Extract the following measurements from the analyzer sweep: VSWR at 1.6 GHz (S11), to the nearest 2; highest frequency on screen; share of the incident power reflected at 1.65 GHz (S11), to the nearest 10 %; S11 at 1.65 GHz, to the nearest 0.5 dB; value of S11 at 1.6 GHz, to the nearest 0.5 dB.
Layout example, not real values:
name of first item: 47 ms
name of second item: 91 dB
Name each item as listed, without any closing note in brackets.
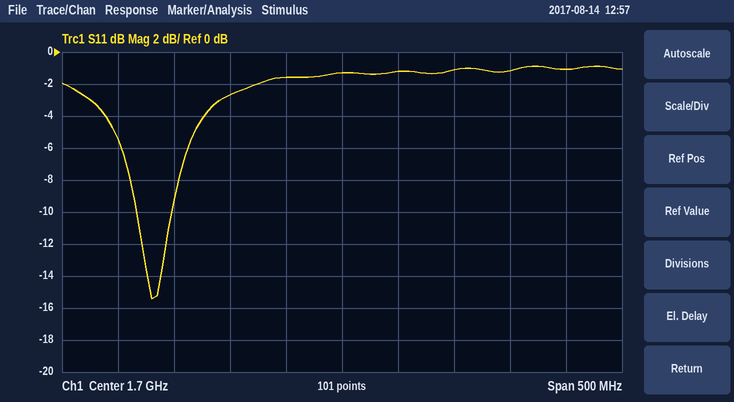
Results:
VSWR at 1.6 GHz (S11), to the nearest 2: 6
highest frequency on screen: 1.95 GHz
share of the incident power reflected at 1.65 GHz (S11), to the nearest 10 %: 70 %
S11 at 1.65 GHz, to the nearest 0.5 dB: -1.5 dB
value of S11 at 1.6 GHz, to the nearest 0.5 dB: -2.5 dB
